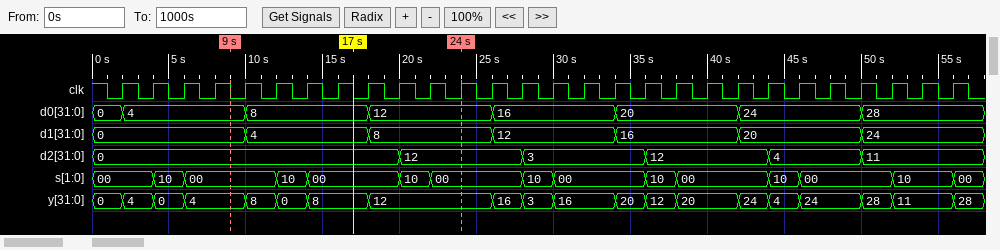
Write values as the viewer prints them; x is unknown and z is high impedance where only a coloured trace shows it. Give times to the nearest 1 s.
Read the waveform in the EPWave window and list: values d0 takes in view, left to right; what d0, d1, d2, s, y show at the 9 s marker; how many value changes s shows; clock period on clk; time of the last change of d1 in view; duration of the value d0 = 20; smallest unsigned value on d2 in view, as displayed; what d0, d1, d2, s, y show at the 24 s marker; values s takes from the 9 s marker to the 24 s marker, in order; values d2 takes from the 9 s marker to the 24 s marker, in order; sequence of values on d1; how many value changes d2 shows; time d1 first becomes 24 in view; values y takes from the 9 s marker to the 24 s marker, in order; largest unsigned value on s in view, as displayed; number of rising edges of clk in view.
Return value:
0, 4, 8, 12, 16, 20, 24, 28
d0=4, d1=0, d2=0, s=00, y=4
14
2 s
50 s
8 s
0
d0=12, d1=8, d2=12, s=00, y=12
00, 10, 00, 10, 00
0, 12
0, 4, 8, 12, 16, 20, 24
5
50 s
4, 8, 0, 8, 12
10
28
